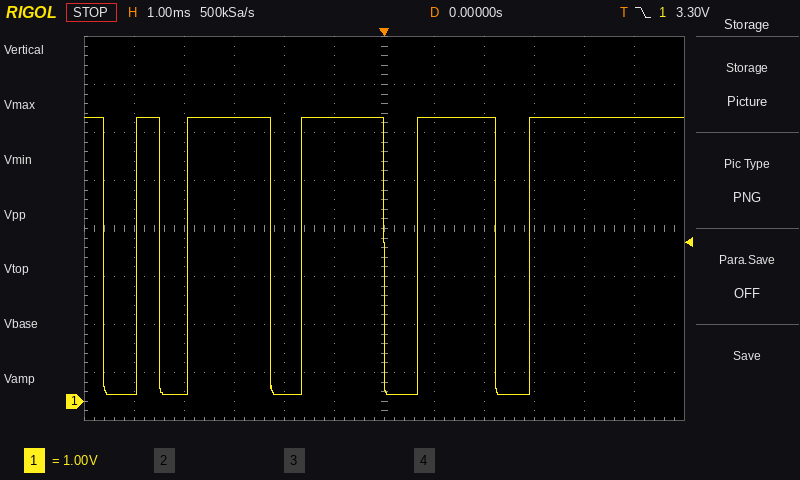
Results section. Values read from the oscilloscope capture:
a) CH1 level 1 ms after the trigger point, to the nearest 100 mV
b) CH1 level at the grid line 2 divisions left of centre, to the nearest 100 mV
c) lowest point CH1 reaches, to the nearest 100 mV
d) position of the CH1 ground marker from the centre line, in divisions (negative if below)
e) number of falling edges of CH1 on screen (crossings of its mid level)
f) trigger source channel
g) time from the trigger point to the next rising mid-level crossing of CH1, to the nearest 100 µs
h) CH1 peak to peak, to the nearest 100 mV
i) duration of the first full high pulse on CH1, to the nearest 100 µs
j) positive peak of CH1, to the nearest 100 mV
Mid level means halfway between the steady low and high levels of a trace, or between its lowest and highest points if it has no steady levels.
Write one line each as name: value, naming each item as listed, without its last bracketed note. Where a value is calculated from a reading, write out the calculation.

CH1 level 1 ms after the trigger point, to the nearest 100 mV: 5.9 V
CH1 level at the grid line 2 divisions left of centre, to the nearest 100 mV: 100 mV
lowest point CH1 reaches, to the nearest 100 mV: 100 mV
position of the CH1 ground marker from the centre line, in divisions: -3.6 div
number of falling edges of CH1 on screen: 5
trigger source channel: CH1
time from the trigger point to the next rising mid-level crossing of CH1, to the nearest 100 µs: 700 µs
CH1 peak to peak, to the nearest 100 mV: 5.9 V − (100 mV) = 5.8 V
duration of the first full high pulse on CH1, to the nearest 100 µs: 500 µs
positive peak of CH1, to the nearest 100 mV: 5.9 V
